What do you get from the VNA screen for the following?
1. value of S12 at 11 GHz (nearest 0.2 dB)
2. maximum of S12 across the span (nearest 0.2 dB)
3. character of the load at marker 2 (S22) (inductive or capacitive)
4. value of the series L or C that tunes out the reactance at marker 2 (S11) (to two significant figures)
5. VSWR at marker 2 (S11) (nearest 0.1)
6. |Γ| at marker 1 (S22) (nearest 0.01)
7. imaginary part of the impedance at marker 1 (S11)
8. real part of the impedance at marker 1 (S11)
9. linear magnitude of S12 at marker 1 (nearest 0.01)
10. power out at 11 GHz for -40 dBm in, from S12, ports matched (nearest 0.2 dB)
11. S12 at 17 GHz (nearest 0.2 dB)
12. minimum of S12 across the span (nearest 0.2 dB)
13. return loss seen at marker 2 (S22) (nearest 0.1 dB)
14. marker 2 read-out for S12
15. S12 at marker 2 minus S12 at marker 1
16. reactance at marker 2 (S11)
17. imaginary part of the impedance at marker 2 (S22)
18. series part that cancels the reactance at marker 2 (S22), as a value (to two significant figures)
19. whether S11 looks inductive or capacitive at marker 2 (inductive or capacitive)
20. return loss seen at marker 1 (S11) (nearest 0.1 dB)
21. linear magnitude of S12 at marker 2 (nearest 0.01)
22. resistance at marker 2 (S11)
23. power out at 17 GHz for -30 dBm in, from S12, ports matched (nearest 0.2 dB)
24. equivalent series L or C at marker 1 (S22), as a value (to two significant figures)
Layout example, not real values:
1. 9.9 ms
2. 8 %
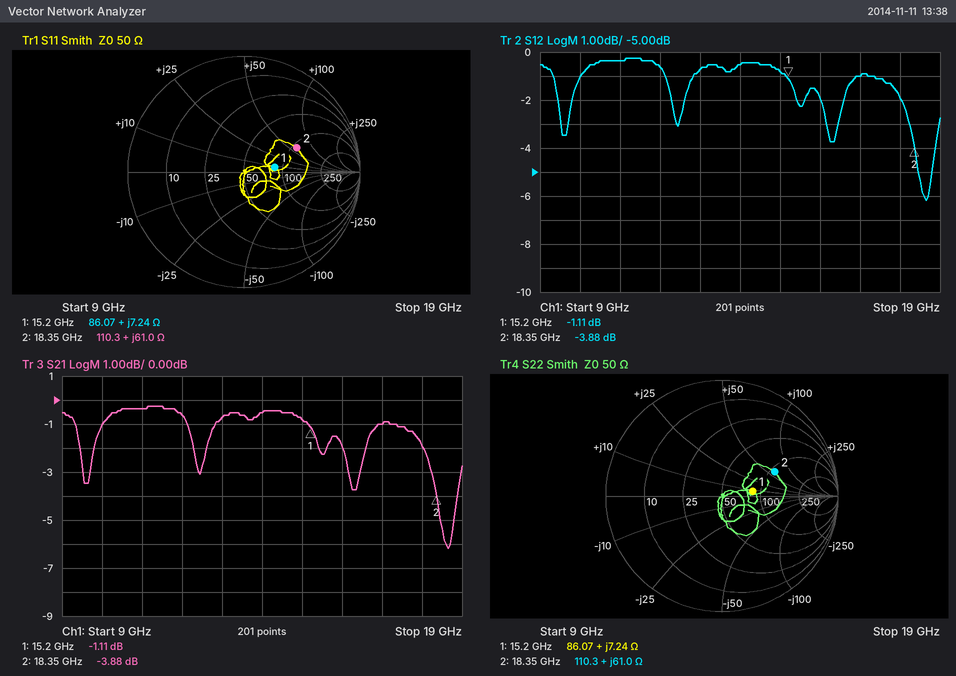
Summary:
1. -0.4 dB
2. -0.2 dB
3. inductive
4. 140 fF
5. 3.0
6. 0.27
7. +7.24 Ω
8. 86.07 Ω
9. 0.88
10. -40.4 dBm
11. -1.0 dB
12. -6.2 dB
13. 6.0 dB
14. -3.88 dB
15. -2.77 dB
16. +61.0 Ω
17. +61.0 Ω
18. 140 fF
19. inductive
20. 11.4 dB
21. 0.64
22. 110.3 Ω
23. -31.0 dBm
24. 76 pH
